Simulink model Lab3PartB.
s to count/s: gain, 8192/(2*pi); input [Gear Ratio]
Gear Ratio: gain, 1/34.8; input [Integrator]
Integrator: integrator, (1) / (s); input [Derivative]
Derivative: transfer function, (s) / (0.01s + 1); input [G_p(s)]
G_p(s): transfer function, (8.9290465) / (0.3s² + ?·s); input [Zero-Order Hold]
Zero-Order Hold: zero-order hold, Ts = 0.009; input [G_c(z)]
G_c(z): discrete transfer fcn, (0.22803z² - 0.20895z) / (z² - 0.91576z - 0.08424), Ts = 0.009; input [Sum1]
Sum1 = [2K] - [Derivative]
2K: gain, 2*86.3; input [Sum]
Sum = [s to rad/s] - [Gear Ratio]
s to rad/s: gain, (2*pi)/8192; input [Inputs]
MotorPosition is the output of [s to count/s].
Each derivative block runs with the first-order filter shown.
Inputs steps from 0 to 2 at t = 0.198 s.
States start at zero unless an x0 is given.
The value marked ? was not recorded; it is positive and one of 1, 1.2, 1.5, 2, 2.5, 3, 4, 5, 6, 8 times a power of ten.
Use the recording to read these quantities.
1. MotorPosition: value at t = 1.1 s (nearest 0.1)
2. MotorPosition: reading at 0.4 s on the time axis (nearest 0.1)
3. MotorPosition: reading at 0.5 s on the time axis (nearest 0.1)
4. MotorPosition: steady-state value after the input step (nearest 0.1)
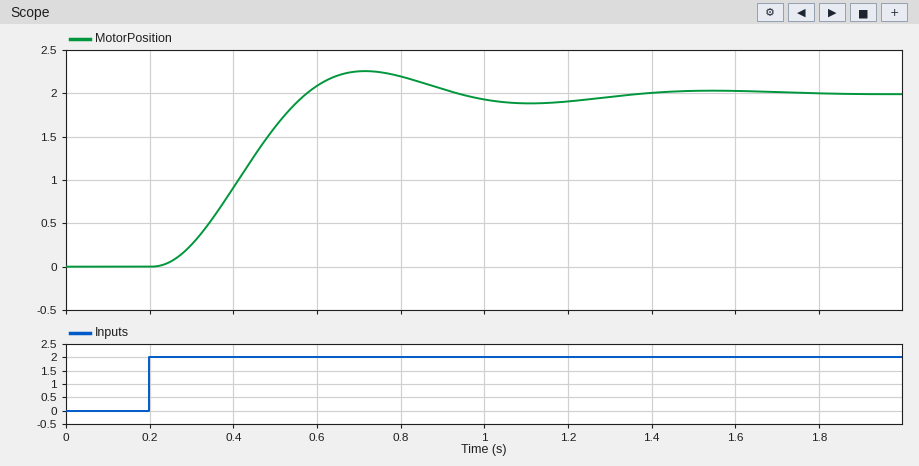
1.9
0.9
1.6
2.0
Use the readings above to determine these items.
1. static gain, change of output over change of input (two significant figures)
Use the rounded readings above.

1.0
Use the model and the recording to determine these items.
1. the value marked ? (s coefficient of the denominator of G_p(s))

1.5
